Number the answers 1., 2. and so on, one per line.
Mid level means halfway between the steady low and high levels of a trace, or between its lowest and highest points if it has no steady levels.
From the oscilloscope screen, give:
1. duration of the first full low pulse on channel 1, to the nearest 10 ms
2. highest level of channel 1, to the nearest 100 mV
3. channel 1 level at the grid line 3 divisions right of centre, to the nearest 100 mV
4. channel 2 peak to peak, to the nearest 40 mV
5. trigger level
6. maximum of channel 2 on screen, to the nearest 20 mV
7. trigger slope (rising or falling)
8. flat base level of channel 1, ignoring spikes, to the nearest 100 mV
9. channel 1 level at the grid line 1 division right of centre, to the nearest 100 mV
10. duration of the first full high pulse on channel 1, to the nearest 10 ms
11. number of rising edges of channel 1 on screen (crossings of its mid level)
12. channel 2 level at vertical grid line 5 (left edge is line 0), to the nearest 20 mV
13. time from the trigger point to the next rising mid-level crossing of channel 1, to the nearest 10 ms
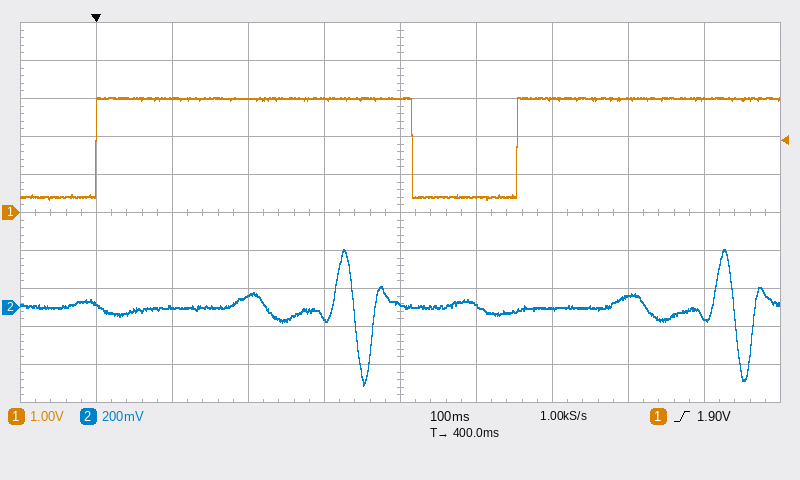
1. 140 ms
2. 3.0 V
3. 3.0 V
4. 720 mV
5. 1.90 V
6. 300 mV
7. rising
8. 400 mV
9. 400 mV
10. 420 ms
11. 2
12. 20 mV
13. 550 ms
